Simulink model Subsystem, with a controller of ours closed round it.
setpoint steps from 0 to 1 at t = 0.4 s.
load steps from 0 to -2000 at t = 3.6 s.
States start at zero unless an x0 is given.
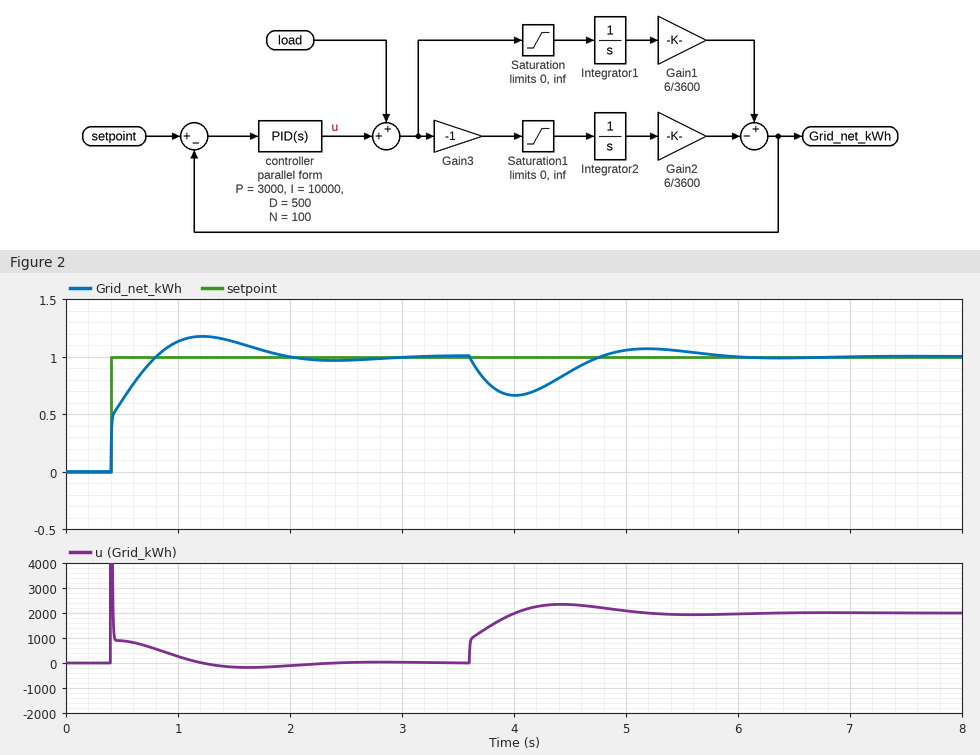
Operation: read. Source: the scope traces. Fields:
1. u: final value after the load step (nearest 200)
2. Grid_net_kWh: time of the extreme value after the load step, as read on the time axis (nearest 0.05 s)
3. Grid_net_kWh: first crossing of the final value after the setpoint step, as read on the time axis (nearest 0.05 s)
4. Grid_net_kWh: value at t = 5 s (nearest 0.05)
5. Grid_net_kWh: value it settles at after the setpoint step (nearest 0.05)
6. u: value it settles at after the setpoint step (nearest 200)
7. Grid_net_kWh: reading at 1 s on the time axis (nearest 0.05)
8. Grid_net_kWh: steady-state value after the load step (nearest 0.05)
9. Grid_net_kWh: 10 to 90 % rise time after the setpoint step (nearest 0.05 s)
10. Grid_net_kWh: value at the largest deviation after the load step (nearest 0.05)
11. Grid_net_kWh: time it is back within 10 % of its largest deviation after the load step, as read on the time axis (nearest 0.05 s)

2000
4.00 s
0.80 s
1.05
1.00
0
1.15
1.00
0.30 s
0.65
5.60 s
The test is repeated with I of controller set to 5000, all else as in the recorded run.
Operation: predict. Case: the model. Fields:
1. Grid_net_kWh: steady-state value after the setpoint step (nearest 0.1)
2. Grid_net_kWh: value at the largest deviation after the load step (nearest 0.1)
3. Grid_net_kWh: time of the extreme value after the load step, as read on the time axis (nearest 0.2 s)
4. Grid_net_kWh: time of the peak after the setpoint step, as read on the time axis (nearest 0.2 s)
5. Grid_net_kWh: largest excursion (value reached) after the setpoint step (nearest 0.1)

1.0
0.6
4.2 s
1.4 s
1.1
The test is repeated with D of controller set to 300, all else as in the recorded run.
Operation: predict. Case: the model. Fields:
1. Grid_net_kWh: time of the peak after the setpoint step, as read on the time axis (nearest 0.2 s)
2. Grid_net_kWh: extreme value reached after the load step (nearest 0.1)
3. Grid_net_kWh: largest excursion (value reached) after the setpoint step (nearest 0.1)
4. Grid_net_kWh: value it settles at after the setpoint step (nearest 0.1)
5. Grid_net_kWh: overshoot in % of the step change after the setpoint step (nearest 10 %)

1.2 s
0.6
1.2
1.0
20 %
